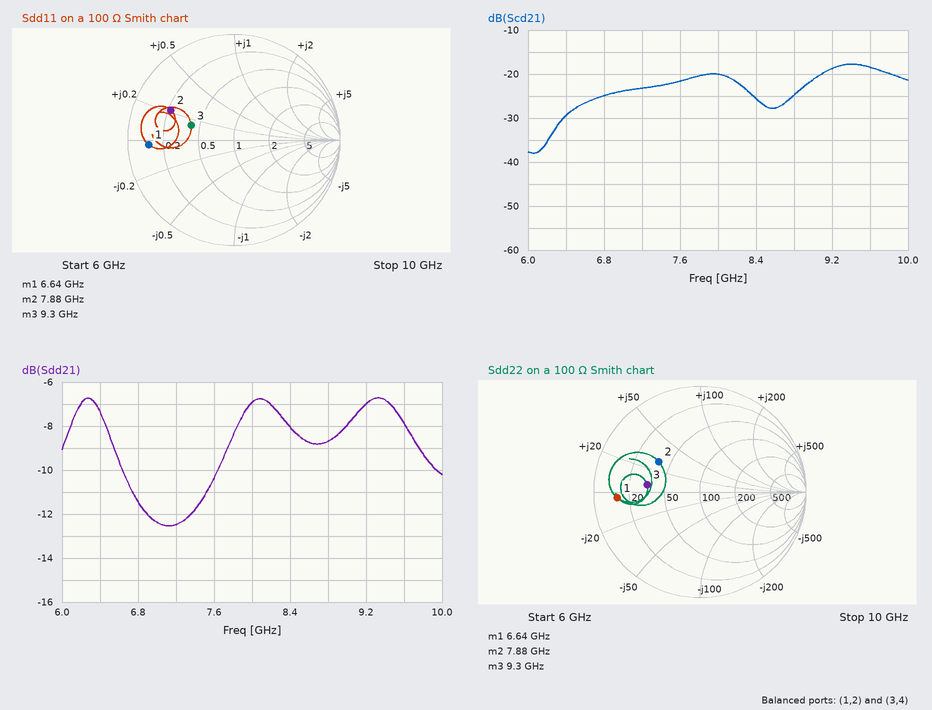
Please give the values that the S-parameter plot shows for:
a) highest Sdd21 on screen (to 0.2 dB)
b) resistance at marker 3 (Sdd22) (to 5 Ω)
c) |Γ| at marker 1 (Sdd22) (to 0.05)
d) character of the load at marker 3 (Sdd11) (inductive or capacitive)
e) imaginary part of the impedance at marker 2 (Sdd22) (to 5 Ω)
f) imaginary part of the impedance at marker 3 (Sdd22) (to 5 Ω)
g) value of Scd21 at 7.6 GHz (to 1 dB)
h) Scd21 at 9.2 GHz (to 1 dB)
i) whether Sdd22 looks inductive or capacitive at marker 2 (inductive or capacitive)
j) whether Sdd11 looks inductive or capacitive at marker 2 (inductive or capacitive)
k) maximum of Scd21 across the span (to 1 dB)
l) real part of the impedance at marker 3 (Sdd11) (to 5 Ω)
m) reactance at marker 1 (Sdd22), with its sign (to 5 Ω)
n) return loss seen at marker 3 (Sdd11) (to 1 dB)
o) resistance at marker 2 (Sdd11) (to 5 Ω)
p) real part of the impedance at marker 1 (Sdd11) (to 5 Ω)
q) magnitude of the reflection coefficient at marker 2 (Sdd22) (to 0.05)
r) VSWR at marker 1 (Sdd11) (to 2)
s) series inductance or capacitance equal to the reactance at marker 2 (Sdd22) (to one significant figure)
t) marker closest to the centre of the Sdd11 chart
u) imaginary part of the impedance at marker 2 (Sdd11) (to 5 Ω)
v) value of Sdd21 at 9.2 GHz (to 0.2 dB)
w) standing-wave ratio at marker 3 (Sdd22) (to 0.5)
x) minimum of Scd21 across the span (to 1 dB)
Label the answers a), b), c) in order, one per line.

a) -6.8 dB
b) 35 Ω
c) 0.80
d) inductive
e) +30 Ω
f) +5 Ω
g) -22 dB
h) -19 dB
i) inductive
j) inductive
k) -18 dB
l) 40 Ω
m) -5 Ω
n) 7 dB
o) 20 Ω
p) 10 Ω
q) 0.50
r) 10
s) 600 pH
t) marker 3
u) +20 Ω
v) -7.0 dB
w) 3.0
x) -38 dB
